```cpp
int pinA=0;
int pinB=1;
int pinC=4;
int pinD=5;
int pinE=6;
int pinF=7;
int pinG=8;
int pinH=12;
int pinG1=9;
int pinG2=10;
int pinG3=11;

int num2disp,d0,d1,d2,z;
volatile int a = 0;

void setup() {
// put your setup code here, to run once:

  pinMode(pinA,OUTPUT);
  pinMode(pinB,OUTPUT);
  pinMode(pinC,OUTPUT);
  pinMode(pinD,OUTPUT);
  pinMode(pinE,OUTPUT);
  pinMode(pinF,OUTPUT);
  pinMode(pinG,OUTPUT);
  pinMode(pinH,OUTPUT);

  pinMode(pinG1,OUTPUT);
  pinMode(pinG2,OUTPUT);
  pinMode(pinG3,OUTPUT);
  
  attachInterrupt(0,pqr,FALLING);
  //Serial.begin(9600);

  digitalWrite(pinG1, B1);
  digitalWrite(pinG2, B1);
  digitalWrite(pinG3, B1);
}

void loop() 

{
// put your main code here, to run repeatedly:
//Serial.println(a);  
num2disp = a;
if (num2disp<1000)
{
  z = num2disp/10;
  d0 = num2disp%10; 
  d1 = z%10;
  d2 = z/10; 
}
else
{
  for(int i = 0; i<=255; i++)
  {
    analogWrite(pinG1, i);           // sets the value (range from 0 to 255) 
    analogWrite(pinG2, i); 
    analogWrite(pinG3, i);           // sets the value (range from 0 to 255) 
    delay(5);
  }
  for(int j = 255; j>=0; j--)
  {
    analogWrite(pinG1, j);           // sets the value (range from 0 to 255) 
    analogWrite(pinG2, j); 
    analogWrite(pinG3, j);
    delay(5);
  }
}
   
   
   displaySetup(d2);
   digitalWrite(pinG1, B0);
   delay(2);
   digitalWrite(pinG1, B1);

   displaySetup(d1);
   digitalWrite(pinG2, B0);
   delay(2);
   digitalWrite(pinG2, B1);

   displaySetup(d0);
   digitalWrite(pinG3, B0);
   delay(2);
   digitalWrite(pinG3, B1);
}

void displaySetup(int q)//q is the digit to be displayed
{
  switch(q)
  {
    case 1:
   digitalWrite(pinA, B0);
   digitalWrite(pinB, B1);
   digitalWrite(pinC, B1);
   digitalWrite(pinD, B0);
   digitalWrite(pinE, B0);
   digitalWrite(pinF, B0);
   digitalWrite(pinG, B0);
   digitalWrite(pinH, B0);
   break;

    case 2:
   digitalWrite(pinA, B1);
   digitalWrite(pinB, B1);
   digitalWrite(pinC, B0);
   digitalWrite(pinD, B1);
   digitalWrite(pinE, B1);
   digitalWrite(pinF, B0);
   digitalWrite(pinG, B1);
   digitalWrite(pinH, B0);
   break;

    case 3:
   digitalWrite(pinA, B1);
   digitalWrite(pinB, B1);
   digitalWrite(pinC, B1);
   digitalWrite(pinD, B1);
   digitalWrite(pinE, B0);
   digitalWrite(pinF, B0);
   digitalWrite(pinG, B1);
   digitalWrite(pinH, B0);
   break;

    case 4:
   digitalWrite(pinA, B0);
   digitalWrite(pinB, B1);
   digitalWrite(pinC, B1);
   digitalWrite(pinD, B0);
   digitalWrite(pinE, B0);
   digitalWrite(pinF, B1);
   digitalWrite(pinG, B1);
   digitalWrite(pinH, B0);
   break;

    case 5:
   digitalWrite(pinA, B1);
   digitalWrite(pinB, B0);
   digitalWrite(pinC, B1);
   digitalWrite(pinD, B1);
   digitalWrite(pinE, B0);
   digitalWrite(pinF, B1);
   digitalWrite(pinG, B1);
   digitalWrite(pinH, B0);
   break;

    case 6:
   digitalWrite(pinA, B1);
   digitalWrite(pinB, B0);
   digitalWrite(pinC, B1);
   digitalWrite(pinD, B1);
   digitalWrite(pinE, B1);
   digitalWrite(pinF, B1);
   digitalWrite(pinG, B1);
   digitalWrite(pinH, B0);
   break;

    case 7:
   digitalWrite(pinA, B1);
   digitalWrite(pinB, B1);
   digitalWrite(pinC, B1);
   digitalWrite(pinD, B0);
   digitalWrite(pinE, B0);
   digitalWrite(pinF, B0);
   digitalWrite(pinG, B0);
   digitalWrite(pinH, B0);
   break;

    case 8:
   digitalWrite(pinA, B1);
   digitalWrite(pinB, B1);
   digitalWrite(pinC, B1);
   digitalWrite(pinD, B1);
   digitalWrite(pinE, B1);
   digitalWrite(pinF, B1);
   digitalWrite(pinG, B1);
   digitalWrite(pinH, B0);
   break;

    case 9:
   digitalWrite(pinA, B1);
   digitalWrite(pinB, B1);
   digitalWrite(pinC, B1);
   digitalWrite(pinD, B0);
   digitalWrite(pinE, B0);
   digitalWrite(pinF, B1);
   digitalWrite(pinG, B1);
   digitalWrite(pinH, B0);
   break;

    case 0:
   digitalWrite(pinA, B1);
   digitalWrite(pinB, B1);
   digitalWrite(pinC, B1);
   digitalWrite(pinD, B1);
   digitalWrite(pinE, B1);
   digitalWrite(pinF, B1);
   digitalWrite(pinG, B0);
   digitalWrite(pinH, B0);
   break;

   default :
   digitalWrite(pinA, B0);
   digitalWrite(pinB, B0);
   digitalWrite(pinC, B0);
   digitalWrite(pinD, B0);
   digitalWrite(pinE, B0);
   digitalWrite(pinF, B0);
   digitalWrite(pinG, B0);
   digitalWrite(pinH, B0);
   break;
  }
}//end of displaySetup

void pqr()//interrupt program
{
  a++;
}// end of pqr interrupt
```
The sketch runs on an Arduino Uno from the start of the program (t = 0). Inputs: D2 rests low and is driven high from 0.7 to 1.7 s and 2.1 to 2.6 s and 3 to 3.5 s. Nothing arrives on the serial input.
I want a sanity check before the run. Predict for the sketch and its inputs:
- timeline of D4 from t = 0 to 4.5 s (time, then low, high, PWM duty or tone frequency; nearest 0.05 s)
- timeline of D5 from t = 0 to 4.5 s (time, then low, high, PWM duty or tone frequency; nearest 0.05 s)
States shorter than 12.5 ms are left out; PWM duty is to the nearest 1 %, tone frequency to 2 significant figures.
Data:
0 s high; 2.6 s tone 160 Hz; 3.5 s high
0 s high; 1.7 s tone 160 Hz; 2.6 s high
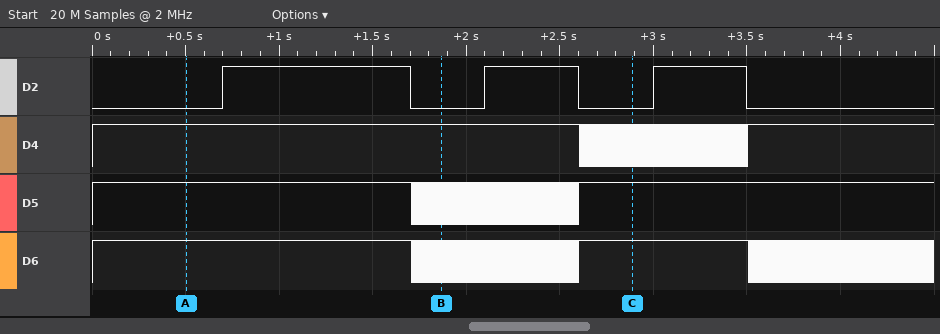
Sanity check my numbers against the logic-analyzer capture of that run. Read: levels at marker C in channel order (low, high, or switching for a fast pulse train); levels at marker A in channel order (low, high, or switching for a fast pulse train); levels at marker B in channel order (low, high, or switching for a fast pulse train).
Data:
D2 low, D4 switching, D5 high, D6 high
D2 low, D4 high, D5 high, D6 high
D2 low, D4 high, D5 switching, D6 switching
